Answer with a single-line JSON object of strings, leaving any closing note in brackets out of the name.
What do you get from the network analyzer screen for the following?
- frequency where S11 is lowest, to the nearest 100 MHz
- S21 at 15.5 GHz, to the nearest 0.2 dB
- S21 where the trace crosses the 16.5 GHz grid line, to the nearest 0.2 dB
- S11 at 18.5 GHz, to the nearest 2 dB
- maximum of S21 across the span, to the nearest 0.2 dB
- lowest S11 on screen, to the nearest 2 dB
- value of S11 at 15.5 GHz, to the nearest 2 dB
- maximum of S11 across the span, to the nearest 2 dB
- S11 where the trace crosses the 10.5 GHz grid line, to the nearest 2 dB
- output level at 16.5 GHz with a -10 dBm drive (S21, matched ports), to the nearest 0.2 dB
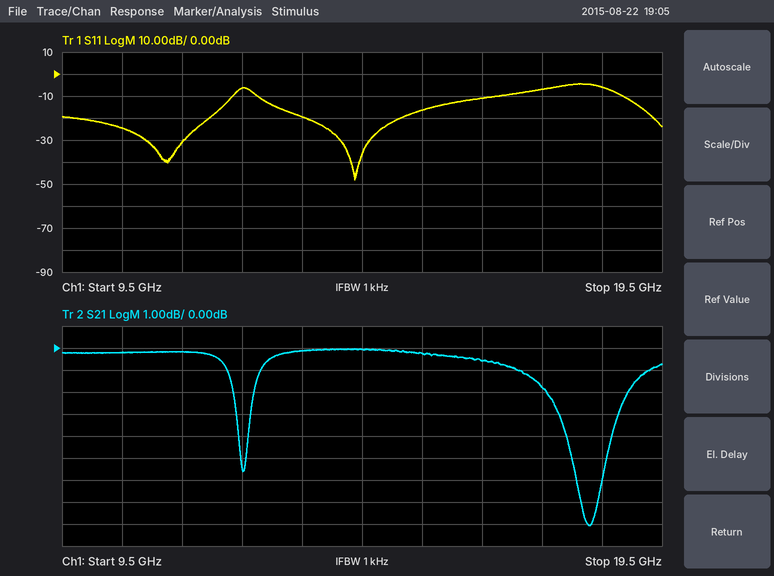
{"frequency where S11 is lowest, to the nearest 100 MHz": "14.4 GHz", "S21 at 15.5 GHz, to the nearest 0.2 dB": "-0.2 dB", "S21 where the trace crosses the 16.5 GHz grid line, to the nearest 0.2 dB": "-0.6 dB", "S11 at 18.5 GHz, to the nearest 2 dB": "-6 dB", "maximum of S21 across the span, to the nearest 0.2 dB": "0.0 dB", "lowest S11 on screen, to the nearest 2 dB": "-48 dB", "value of S11 at 15.5 GHz, to the nearest 2 dB": "-16 dB", "maximum of S11 across the span, to the nearest 2 dB": "-4 dB", "S11 where the trace crosses the 10.5 GHz grid line, to the nearest 2 dB": "-24 dB", "output level at 16.5 GHz with a -10 dBm drive (S21, matched ports), to the nearest 0.2 dB": "-10.6 dBm"}
